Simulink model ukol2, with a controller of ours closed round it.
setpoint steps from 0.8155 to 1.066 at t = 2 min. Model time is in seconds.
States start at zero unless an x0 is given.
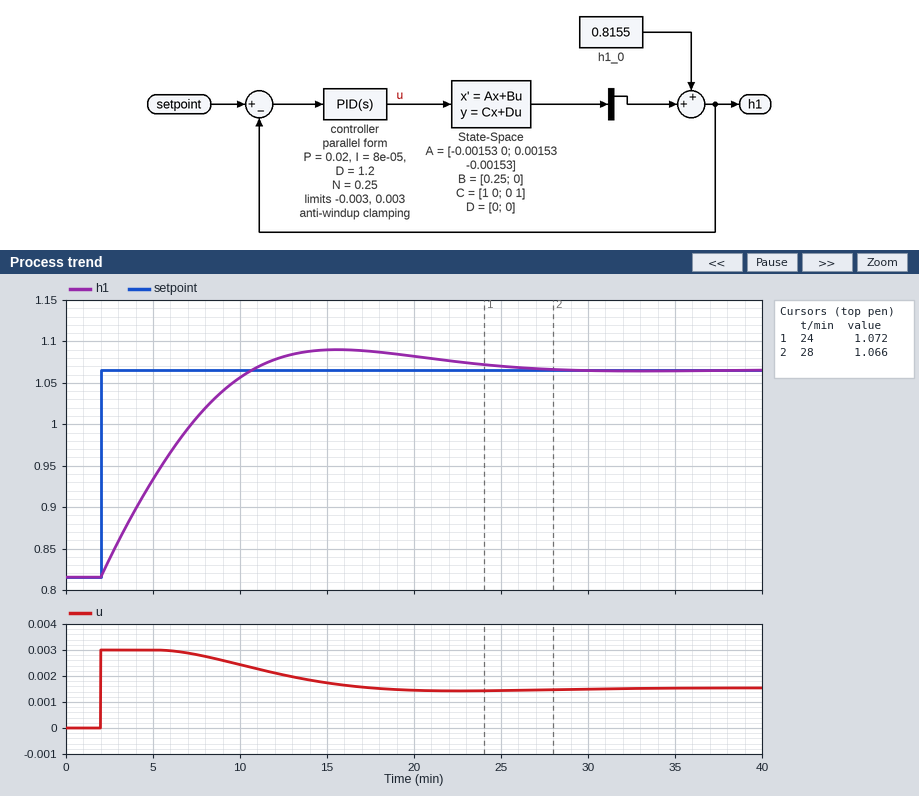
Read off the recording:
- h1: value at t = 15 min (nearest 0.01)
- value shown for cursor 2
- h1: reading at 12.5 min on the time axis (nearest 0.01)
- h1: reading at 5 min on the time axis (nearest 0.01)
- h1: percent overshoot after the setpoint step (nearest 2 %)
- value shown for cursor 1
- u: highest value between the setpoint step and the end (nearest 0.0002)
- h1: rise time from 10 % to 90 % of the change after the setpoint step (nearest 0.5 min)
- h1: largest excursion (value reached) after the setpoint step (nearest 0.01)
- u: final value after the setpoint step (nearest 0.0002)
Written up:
1.09
1.066
1.08
0.93
10 %
1.072
0.0030
6.5 min
1.09
0.0016
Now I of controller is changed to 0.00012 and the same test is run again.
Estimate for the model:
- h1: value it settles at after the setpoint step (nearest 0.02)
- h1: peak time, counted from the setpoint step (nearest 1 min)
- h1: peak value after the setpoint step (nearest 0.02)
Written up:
1.06
12 min
1.10
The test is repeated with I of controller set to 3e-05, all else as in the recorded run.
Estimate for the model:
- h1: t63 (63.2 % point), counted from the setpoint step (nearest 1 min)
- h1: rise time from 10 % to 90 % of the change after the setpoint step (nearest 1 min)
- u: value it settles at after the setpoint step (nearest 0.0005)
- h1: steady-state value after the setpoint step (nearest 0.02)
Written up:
5 min
10 min
0.0015
1.06
